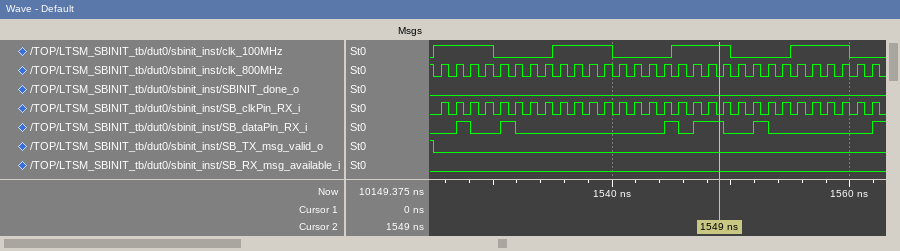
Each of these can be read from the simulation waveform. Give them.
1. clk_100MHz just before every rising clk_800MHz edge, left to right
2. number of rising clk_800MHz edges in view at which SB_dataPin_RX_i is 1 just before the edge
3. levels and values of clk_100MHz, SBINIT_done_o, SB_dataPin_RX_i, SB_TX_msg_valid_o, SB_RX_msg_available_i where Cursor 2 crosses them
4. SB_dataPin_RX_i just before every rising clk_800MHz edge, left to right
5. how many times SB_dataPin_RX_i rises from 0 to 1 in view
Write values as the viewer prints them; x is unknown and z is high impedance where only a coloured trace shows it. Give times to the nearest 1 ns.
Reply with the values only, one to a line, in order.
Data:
1 1 1 1 0 0 0 0 1 1 1 1 0 0 0 0 1 1 1 1 0 0 0 0 1 1 1 1 0 0
6
clk_100MHz=1, SBINIT_done_o=0, SB_dataPin_RX_i=1, SB_TX_msg_valid_o=0, SB_RX_msg_available_i=0
0 0 1 0 0 1 0 0 0 0 0 0 0 0 0 0 1 0 1 1 0 0 1 0 0 0 0 0 0 0
6
